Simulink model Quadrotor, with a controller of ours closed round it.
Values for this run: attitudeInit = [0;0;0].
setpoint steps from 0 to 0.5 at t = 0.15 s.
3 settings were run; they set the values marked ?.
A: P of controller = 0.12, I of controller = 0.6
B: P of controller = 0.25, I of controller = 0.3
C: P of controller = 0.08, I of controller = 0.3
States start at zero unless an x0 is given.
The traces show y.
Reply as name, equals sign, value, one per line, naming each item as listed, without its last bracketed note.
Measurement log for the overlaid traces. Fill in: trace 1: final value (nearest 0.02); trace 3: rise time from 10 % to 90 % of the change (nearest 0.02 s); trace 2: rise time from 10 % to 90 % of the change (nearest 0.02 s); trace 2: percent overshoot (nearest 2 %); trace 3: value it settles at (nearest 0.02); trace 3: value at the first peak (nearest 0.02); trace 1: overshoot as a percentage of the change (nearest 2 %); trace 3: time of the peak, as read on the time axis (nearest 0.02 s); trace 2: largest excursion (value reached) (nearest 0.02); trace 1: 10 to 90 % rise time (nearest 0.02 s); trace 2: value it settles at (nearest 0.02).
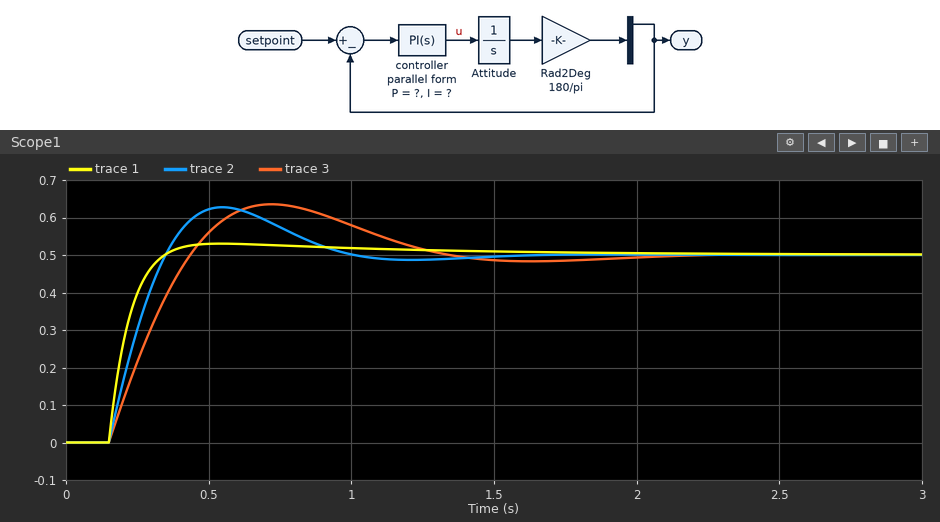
trace 1: final value = 0.50
trace 3: rise time from 10 % to 90 % of the change = 0.22 s
trace 2: rise time from 10 % to 90 % of the change = 0.16 s
trace 2: percent overshoot = 26 %
trace 3: value it settles at = 0.50
trace 3: value at the first peak = 0.64
trace 1: overshoot as a percentage of the change = 6 %
trace 3: time of the peak, as read on the time axis = 0.72 s
trace 2: largest excursion (value reached) = 0.62
trace 1: 10 to 90 % rise time = 0.12 s
trace 2: value it settles at = 0.50
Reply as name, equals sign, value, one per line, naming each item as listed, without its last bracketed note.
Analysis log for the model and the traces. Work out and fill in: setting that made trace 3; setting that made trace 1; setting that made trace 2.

setting that made trace 3 = C
setting that made trace 1 = B
setting that made trace 2 = A
